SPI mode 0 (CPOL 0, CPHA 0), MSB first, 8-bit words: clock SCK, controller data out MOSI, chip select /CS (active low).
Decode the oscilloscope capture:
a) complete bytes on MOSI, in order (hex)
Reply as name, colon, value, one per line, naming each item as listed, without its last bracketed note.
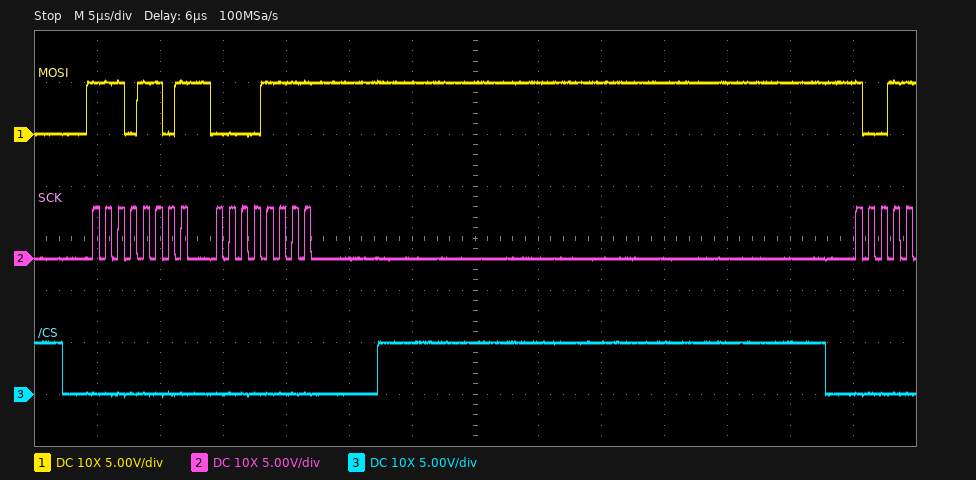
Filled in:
complete bytes on MOSI, in order: 0xED 0x0F
